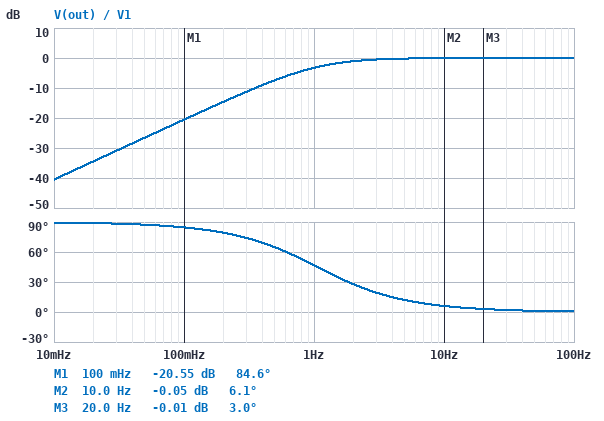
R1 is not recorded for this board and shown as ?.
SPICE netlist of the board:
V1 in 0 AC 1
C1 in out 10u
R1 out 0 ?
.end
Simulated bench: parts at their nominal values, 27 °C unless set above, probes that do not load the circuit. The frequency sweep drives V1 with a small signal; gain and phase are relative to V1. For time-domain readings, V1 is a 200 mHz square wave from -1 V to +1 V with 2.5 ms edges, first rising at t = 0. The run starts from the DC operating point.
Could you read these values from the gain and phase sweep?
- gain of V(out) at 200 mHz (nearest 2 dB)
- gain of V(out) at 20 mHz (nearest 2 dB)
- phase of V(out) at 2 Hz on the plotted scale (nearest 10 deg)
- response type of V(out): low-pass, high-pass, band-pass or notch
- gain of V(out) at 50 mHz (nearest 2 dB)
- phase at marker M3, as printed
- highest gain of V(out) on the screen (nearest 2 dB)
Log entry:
-14 dB
-34 dB
30 deg
high-pass
-26 dB
3.0 deg
0 dB
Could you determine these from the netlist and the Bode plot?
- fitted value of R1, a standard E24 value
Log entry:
15 kΩ
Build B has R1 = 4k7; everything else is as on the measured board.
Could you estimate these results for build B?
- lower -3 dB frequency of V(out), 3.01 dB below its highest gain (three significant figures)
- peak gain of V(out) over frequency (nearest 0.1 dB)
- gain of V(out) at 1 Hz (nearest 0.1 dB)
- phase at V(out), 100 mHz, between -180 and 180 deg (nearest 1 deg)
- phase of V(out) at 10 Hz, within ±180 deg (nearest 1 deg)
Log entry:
3.39 Hz
0 dB
-11.0 dB
88 deg
19 deg
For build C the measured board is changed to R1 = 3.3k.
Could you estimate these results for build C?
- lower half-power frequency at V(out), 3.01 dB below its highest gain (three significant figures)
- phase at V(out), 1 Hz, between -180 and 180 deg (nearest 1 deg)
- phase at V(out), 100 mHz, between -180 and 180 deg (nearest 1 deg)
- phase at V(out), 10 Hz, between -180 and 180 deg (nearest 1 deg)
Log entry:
4.82 Hz
78 deg
89 deg
26 deg
